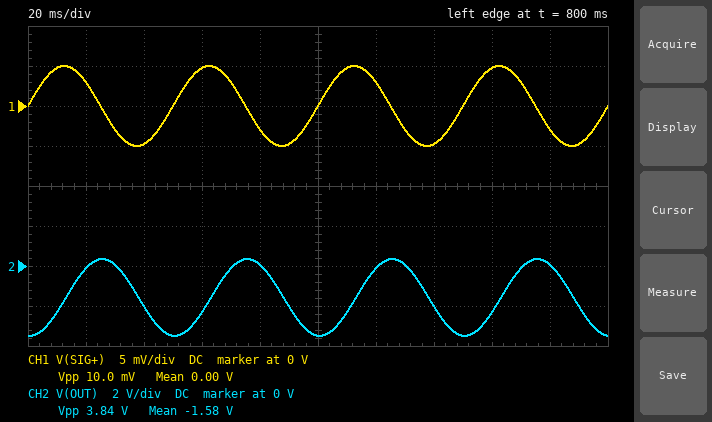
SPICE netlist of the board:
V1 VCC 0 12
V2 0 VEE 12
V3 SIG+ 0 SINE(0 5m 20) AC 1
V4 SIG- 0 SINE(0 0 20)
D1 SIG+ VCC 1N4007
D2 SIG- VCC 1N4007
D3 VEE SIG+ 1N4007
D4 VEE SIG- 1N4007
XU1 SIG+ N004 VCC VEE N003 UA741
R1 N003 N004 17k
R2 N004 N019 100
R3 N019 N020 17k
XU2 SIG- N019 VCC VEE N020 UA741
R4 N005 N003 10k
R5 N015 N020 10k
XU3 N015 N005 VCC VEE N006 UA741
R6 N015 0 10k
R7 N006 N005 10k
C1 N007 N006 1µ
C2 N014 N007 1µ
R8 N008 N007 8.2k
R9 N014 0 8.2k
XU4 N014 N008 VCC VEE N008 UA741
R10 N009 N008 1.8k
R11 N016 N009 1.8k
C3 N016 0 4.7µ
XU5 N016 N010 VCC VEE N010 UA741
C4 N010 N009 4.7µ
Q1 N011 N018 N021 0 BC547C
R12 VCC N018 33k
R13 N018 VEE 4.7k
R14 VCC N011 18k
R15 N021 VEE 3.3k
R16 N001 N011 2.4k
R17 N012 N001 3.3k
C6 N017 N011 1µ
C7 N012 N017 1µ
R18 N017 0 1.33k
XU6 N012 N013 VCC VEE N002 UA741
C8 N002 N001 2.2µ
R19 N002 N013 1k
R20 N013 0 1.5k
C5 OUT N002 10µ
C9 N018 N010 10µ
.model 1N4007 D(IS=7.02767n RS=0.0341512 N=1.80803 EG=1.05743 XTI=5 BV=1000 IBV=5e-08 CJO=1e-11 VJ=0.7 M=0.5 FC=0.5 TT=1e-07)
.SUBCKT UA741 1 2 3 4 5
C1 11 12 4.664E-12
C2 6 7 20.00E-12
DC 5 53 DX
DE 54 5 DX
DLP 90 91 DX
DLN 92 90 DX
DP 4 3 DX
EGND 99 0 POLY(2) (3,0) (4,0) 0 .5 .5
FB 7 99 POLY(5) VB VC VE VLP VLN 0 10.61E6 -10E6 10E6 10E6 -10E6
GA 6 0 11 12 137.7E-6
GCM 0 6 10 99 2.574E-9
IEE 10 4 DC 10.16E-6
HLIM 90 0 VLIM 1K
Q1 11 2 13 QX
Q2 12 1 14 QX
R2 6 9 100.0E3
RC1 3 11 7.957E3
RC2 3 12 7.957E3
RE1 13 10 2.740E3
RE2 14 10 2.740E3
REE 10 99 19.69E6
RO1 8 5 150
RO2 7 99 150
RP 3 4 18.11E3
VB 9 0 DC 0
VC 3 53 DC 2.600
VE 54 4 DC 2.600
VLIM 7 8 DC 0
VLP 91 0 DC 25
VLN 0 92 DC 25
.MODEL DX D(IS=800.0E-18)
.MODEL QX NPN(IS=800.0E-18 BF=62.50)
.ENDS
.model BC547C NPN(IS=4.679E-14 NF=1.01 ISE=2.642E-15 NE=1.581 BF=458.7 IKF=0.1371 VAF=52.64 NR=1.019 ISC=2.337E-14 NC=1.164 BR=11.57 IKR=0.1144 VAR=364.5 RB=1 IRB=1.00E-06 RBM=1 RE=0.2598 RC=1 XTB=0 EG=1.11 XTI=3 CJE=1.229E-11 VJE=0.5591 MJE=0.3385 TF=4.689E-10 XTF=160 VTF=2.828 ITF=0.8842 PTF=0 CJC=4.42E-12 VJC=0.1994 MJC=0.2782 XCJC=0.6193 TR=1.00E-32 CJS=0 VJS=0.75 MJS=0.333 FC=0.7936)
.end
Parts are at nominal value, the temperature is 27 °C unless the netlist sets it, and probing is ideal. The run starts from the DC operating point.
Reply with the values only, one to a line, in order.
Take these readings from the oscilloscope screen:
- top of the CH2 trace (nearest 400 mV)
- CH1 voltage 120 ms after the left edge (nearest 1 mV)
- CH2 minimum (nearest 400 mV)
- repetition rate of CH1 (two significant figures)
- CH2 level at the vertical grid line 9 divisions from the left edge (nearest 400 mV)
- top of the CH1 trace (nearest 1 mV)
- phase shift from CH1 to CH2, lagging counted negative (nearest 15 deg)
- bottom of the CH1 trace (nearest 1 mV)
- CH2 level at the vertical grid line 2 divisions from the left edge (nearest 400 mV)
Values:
400 mV
3 mV
-3.6 V
20 Hz
0 V
5 mV
-90 deg
-5 mV
-2.0 V
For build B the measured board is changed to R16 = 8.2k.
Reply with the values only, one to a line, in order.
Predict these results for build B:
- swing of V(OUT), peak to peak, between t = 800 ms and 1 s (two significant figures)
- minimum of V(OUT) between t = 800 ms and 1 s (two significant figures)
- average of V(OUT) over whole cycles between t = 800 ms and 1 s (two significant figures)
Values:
12 V
-7.4 V
-1.6 V
